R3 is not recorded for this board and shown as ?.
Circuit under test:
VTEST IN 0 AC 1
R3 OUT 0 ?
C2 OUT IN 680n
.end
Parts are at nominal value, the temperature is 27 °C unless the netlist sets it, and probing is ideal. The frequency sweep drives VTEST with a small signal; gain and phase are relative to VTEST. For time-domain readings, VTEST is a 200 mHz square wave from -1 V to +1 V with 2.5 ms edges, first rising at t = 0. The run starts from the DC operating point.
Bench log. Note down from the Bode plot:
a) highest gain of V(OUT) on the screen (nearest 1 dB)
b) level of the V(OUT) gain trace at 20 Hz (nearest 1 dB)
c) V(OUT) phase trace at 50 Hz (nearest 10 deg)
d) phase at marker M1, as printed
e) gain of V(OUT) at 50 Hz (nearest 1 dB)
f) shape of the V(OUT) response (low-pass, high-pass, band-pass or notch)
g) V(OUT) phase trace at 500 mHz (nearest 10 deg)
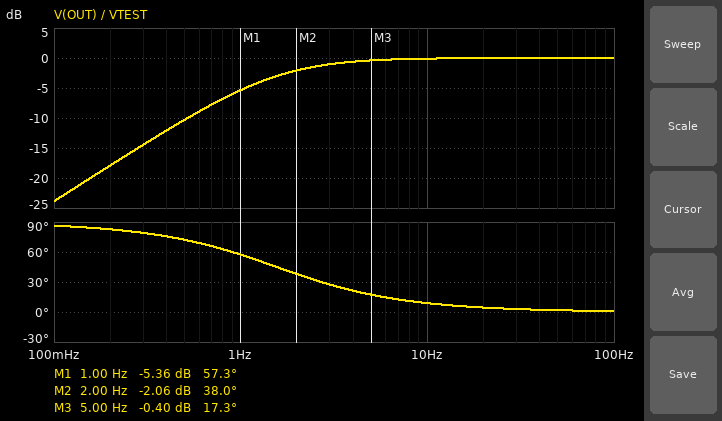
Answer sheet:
0 dB
0 dB
0 deg
57.3 deg
0 dB
high-pass
70 deg
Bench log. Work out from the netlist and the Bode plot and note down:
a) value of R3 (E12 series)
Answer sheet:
150 kΩ
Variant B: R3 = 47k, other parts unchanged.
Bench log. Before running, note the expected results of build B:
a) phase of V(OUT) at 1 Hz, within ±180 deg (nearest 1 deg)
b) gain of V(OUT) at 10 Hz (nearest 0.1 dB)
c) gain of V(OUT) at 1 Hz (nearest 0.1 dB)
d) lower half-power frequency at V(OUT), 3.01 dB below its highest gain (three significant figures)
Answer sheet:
79 deg
-1.0 dB
-14.1 dB
4.98 Hz
